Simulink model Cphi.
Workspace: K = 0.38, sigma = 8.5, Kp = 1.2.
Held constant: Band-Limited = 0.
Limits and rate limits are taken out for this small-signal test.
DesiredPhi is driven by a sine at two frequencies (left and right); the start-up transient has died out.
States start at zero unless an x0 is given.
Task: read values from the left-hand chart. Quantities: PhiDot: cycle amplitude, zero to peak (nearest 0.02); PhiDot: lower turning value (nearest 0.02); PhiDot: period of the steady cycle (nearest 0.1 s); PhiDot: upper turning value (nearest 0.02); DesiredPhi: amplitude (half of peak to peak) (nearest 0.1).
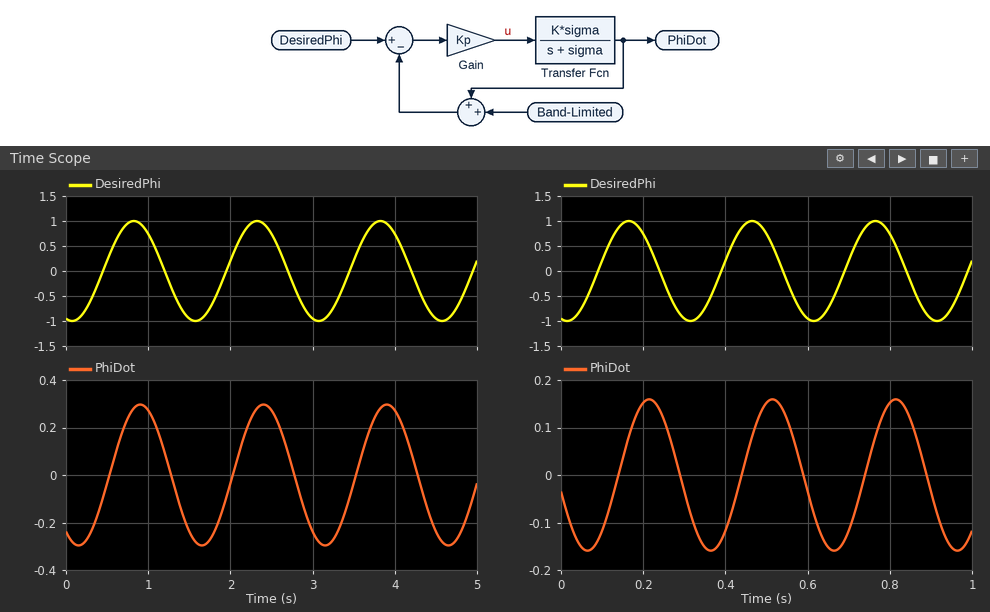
0.30
-0.30
1.5 s
0.30
1.0
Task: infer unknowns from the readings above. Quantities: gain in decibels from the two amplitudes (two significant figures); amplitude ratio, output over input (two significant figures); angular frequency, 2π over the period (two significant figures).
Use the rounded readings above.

-10 dB
0.30
4.2 rad/s
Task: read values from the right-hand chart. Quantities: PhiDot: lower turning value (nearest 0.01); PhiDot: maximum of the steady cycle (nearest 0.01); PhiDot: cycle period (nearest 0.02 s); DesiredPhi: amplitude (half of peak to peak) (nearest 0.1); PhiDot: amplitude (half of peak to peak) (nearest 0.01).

-0.16
0.16
0.30 s
1.0
0.16
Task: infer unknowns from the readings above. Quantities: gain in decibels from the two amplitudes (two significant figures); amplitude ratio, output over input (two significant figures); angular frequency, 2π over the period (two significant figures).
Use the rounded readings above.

-16 dB
0.16
21 rad/s
